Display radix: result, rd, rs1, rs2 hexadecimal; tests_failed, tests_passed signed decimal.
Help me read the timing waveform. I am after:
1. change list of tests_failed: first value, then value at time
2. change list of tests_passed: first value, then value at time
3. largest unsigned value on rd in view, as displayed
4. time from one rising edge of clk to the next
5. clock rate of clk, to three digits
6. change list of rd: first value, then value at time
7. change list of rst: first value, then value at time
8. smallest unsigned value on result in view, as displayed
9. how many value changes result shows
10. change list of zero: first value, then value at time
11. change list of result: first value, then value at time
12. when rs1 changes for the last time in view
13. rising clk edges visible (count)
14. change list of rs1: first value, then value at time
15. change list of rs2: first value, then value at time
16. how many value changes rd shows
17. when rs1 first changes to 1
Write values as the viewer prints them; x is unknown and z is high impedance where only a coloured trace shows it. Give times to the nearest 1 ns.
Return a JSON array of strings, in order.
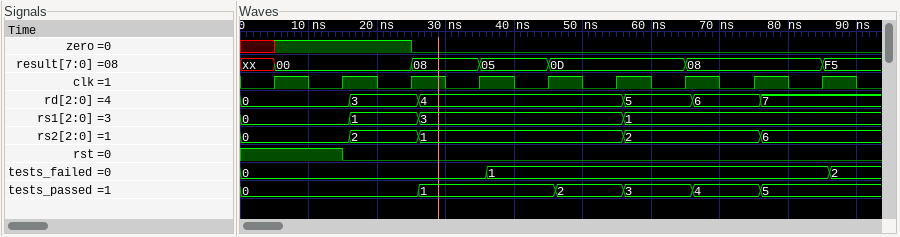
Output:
["0, 1 at 36 ns, 2 at 86 ns", "0, 1 at 26 ns, 2 at 46 ns, 3 at 56 ns, 4 at 66 ns, 5 at 76 ns", "7", "10 ns", "100 MHz", "0, 3 at 16 ns, 4 at 26 ns, 5 at 56 ns, 6 at 66 ns, 7 at 76 ns", "1, 0 at 15 ns", "00", "6", "x, 1 at 5 ns, 0 at 25 ns", "xx, 00 at 5 ns, 08 at 25 ns, 05 at 35 ns, 0D at 45 ns, 08 at 65 ns, F5 at 85 ns", "56 ns", "9", "0, 1 at 16 ns, 3 at 26 ns, 1 at 56 ns", "0, 2 at 16 ns, 1 at 26 ns, 2 at 56 ns, 6 at 76 ns", "5", "16 ns"]
